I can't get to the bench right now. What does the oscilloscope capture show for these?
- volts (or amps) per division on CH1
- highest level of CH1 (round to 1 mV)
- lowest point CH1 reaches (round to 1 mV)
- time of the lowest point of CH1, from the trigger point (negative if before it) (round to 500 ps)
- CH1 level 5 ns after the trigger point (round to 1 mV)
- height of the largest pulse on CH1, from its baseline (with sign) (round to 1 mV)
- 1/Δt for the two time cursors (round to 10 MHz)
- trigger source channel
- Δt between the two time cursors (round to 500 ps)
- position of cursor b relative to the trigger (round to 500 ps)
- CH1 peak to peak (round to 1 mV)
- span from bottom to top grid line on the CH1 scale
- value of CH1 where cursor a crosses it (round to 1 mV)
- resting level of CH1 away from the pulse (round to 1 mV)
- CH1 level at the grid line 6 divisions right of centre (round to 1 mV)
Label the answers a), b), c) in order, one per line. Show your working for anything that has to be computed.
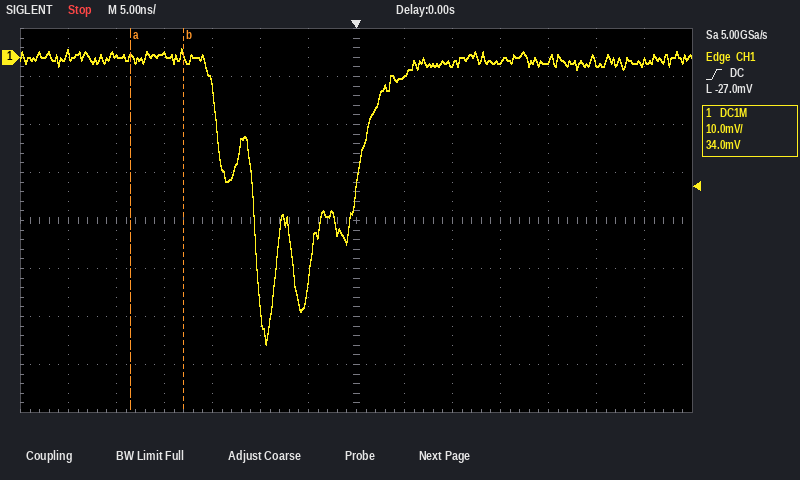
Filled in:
a) 10 mV
b) 2 mV
c) -60 mV
d) -9.5 ns
e) -4 mV
f) -60 mV − (-1 mV) = -59 mV
g) 1 / 5.5 ns ≈ 180 MHz
h) CH1
i) 5.5 ns
j) -18.0 ns
k) 2 mV − (-60 mV) = 62 mV
l) 80 mV
m) 0 mV
n) -1 mV
o) -1 mV
